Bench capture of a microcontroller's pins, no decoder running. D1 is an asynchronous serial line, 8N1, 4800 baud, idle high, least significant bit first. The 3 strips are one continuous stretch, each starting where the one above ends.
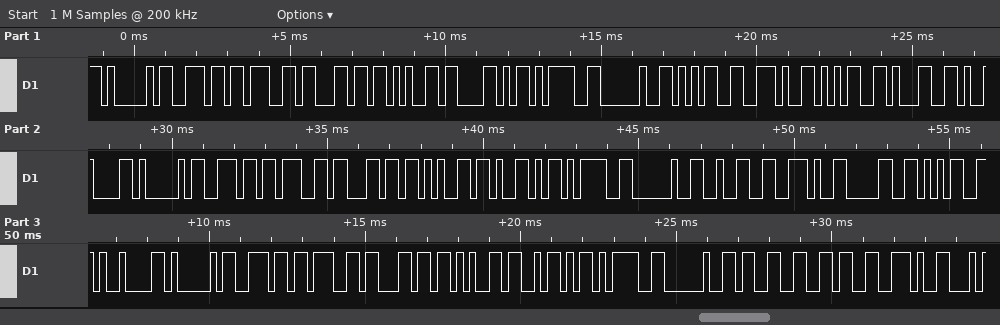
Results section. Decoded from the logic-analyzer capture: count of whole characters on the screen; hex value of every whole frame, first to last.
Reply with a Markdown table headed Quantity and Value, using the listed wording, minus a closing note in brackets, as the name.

| Quantity | Value |
|---|---|
| count of whole characters on the screen | 37 |
| hex value of every whole frame, first to last | 41 6E 67 6C 65 58 3D 20 35 2E 35 31 09 41 6E 67 6C 65 59 3D 20 32 2E 30 35 09 41 6E 67 6C 65 5A 3D 20 33 36 2E |
